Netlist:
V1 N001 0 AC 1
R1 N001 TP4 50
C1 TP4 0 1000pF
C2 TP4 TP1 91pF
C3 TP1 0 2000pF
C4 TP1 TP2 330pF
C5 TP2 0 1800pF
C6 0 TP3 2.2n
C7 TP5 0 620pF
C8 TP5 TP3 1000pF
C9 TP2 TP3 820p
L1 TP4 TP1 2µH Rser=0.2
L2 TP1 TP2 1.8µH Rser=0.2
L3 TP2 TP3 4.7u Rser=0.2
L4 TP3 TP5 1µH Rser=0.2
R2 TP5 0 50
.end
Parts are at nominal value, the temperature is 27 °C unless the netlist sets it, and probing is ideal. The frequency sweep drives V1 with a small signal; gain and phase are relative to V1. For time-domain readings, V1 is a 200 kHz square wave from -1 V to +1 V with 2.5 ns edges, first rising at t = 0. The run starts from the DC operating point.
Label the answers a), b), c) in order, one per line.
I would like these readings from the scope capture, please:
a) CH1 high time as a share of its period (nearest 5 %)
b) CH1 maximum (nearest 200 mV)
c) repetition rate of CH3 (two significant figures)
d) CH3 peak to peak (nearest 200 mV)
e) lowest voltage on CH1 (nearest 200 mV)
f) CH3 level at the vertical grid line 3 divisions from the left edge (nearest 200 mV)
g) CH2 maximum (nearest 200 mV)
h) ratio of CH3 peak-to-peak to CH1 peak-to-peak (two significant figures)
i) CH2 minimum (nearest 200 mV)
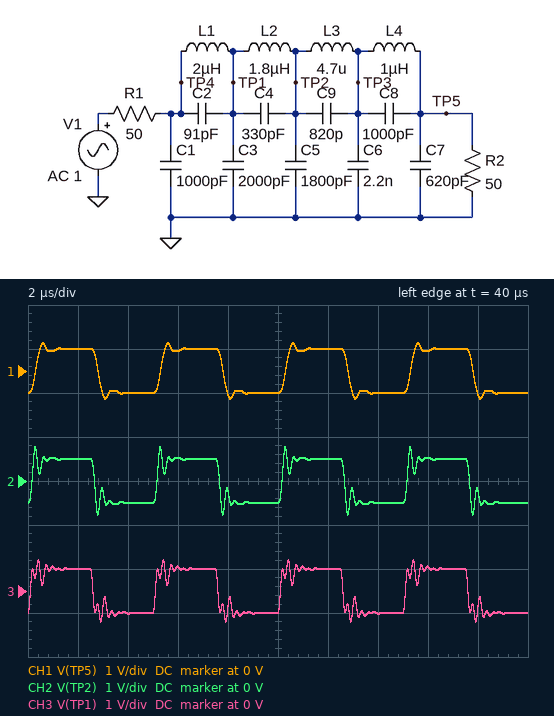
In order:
a) 50 %
b) 600 mV
c) 200 kHz
d) 1.4 V
e) -600 mV
f) 600 mV
g) 800 mV
h) 1.1
i) -800 mV
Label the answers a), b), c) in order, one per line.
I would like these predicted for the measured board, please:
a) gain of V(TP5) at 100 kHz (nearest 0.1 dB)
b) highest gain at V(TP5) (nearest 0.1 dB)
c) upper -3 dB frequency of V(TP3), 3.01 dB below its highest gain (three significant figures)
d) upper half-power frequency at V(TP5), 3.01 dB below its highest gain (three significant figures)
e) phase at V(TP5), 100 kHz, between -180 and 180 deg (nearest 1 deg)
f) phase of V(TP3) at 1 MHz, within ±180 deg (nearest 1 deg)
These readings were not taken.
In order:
a) -6.1 dB
b) -6.1 dB
c) 1.54 MHz
d) 1.57 MHz
e) -10 deg
f) -97 deg
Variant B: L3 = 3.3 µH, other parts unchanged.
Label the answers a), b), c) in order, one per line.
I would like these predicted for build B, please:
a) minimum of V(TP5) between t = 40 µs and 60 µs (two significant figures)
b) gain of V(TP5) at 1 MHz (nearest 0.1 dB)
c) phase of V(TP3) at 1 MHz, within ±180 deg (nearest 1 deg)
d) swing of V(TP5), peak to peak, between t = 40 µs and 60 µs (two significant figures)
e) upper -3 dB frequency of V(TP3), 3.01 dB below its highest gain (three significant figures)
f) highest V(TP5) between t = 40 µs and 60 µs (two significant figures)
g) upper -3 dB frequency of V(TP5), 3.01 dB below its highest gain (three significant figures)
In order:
a) -600 mV
b) -6.5 dB
c) -86 deg
d) 1.2 V
e) 1.87 MHz
f) 600 mV
g) 1.92 MHz
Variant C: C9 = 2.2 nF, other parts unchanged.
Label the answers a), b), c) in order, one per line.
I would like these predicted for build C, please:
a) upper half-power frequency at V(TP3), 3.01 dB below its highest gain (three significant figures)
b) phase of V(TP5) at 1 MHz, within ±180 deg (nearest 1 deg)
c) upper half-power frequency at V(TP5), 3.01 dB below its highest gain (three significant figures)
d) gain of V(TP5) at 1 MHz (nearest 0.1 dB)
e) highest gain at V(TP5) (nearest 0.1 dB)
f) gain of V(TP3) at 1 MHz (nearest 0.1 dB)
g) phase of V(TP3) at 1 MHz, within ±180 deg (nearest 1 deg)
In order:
a) 1.19 MHz
b) -120 deg
c) 1.20 MHz
d) -6.4 dB
e) -6.1 dB
f) -6.5 dB
g) -112 deg
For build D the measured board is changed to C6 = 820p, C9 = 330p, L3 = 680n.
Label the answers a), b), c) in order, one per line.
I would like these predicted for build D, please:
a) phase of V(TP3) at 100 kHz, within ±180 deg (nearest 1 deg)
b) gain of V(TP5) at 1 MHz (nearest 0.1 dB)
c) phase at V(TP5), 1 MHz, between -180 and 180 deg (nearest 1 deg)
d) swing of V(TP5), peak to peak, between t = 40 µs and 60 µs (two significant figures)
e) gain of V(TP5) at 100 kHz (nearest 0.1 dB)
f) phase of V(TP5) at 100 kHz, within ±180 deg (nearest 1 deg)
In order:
a) -7 deg
b) -7.0 dB
c) -70 deg
d) 1.2 V
e) -6.1 dB
f) -8 deg
